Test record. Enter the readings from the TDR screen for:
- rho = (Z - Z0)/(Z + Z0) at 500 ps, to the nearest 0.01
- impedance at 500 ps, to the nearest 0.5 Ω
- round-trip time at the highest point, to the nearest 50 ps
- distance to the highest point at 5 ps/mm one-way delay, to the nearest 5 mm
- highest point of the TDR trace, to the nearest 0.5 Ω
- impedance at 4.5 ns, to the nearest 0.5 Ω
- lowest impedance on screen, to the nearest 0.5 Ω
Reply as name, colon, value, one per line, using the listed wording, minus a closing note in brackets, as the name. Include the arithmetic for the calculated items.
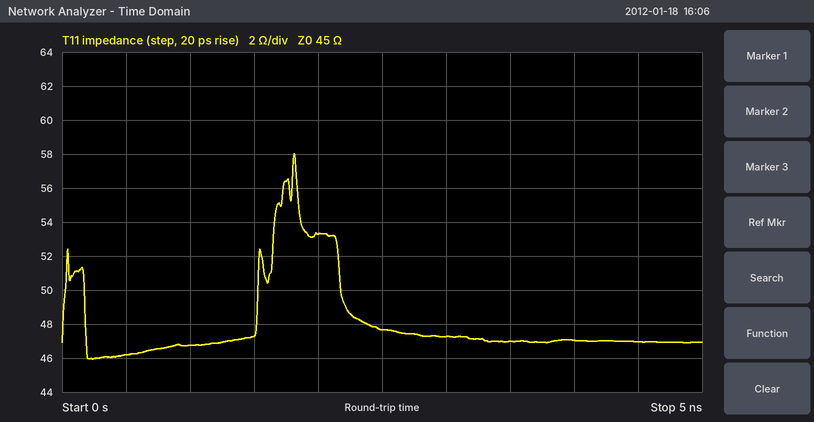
rho = (Z - Z0)/(Z + Z0) at 500 ps, to the nearest 0.01: (46 − 45)/(46 + 45) ≈ +0.01
impedance at 500 ps, to the nearest 0.5 Ω: 46.0 Ω
round-trip time at the highest point, to the nearest 50 ps: 1.80 ns
distance to the highest point at 5 ps/mm one-way delay, to the nearest 5 mm: 1.80 ns / 2 / 5 ps/mm ≈ 180 mm
highest point of the TDR trace, to the nearest 0.5 Ω: 58.0 Ω
impedance at 4.5 ns, to the nearest 0.5 Ω: 47.0 Ω
lowest impedance on screen, to the nearest 0.5 Ω: 46.0 Ω
